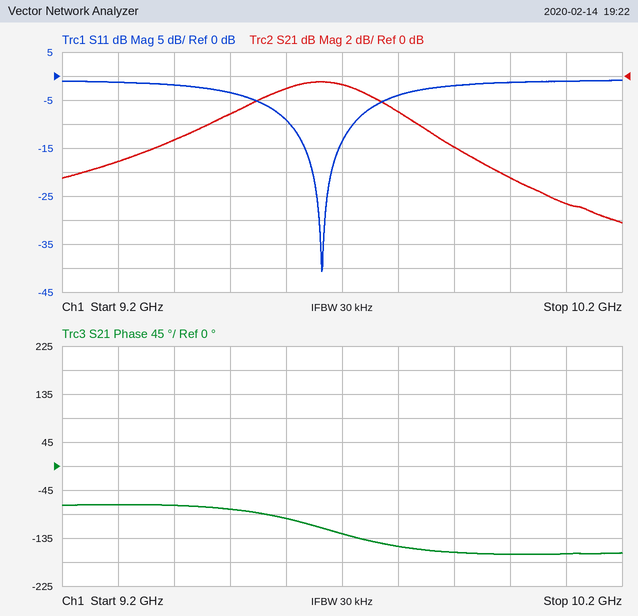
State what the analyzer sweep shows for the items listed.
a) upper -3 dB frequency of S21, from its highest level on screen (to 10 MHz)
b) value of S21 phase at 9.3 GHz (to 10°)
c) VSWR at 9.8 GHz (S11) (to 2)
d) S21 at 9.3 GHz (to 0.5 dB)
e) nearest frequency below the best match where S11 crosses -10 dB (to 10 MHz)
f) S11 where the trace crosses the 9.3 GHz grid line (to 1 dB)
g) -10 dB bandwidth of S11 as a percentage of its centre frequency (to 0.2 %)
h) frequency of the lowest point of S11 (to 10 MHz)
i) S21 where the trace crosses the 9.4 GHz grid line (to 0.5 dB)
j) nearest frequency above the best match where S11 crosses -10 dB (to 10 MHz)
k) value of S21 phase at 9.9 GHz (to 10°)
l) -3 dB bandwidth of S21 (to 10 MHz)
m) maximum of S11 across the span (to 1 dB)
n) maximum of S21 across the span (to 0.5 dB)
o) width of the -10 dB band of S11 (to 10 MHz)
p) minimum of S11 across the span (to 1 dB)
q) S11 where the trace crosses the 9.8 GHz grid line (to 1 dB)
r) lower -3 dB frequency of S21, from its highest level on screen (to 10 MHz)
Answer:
9.82 GHz
-70°
4
-7.0 dB
9.61 GHz
-1 dB
1.2 %
9.66 GHz
-5.5 dB
9.72 GHz
-160°
330 MHz
-1 dB
-0.5 dB
110 MHz
-41 dB
-4 dB
9.49 GHz
